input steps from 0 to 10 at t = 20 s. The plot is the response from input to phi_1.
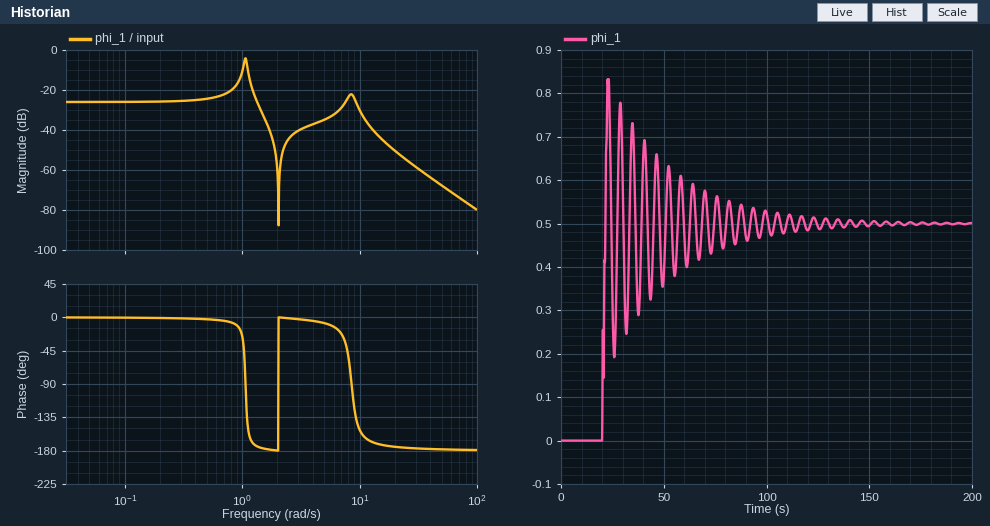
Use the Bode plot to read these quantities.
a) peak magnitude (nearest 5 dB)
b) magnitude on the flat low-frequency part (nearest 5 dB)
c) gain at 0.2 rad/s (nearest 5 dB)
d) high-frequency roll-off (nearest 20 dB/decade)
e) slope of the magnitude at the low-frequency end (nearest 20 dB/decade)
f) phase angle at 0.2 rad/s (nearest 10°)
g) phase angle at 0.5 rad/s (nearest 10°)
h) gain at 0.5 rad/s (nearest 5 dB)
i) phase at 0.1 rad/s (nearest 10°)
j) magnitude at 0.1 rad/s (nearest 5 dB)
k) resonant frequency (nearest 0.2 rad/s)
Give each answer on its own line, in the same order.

-5 dB
-25 dB
-25 dB
-40 dB/decade
0 dB/decade
0°
0°
-25 dB
0°
-25 dB
1.0 rad/s
